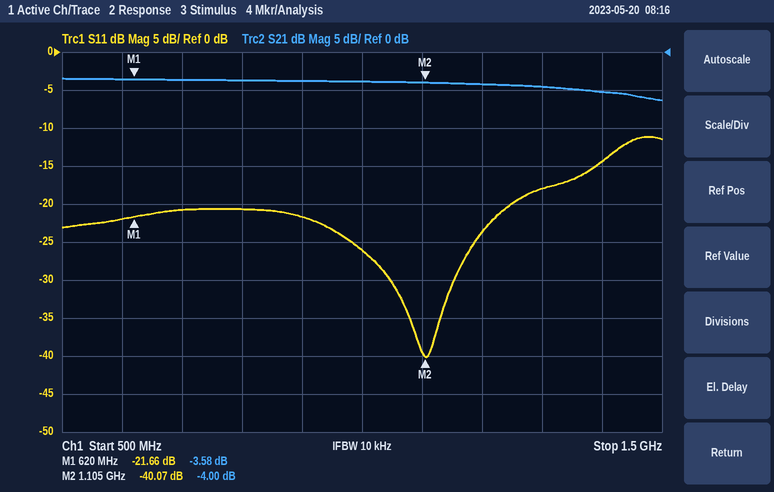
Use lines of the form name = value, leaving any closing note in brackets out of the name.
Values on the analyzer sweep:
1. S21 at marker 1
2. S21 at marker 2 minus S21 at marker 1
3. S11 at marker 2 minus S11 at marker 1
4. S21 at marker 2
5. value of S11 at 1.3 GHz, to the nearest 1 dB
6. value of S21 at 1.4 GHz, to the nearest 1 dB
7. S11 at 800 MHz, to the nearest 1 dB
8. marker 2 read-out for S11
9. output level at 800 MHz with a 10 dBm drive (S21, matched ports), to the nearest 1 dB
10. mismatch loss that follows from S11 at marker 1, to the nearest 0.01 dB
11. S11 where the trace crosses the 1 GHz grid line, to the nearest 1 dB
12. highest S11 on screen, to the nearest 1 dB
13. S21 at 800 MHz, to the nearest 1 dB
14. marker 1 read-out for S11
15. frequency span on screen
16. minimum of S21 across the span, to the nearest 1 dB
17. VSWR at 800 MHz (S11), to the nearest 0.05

S21 at marker 1 = -3.58 dB
S21 at marker 2 minus S21 at marker 1 = -0.42 dB
S11 at marker 2 minus S11 at marker 1 = -18.41 dB
S21 at marker 2 = -4.00 dB
value of S11 at 1.3 GHz, to the nearest 1 dB = -18 dB
value of S21 at 1.4 GHz, to the nearest 1 dB = -5 dB
S11 at 800 MHz, to the nearest 1 dB = -21 dB
marker 2 read-out for S11 = -40.07 dB
output level at 800 MHz with a 10 dBm drive (S21, matched ports), to the nearest 1 dB = 6 dBm
mismatch loss that follows from S11 at marker 1, to the nearest 0.01 dB = 0.03 dB
S11 where the trace crosses the 1 GHz grid line, to the nearest 1 dB = -26 dB
highest S11 on screen, to the nearest 1 dB = -11 dB
S21 at 800 MHz, to the nearest 1 dB = -4 dB
marker 1 read-out for S11 = -21.66 dB
frequency span on screen = 1 GHz
minimum of S21 across the span, to the nearest 1 dB = -6 dB
VSWR at 800 MHz (S11), to the nearest 0.05 = 1.20
